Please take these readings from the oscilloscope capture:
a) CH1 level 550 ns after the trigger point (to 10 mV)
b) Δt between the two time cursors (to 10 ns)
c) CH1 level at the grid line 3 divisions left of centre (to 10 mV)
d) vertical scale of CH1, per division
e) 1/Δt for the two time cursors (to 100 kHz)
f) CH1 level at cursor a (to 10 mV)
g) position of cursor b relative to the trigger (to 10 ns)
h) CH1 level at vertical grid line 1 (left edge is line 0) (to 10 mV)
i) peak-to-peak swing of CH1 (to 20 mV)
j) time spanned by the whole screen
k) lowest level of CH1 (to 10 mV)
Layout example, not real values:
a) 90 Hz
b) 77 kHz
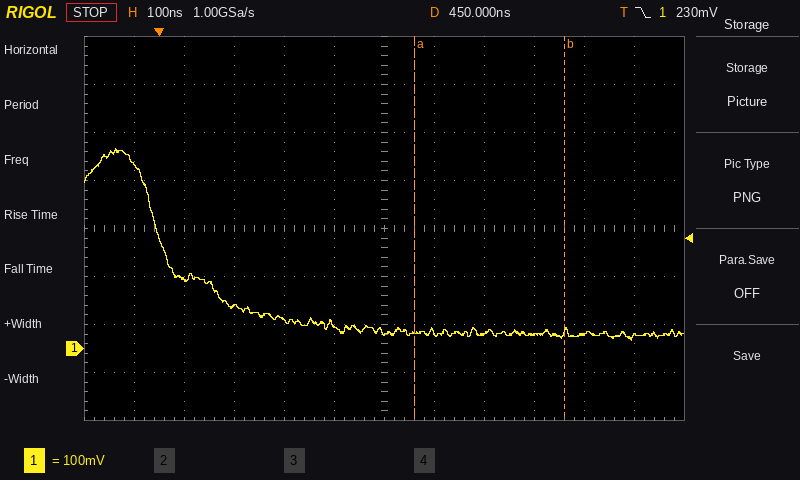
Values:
a) 30 mV
b) 300 ns
c) 90 mV
d) 100 mV
e) 3.3 MHz
f) 30 mV
g) +810 ns
h) 380 mV
i) 400 mV
j) 1.2 µs
k) 20 mV
